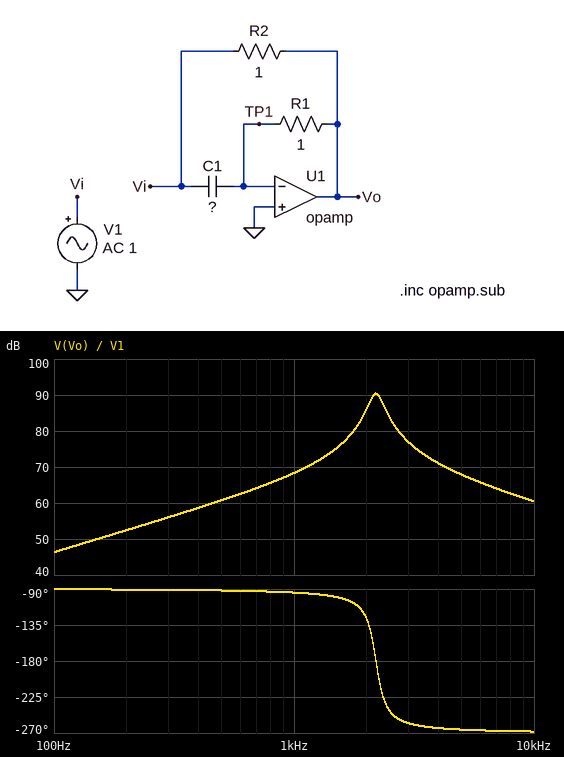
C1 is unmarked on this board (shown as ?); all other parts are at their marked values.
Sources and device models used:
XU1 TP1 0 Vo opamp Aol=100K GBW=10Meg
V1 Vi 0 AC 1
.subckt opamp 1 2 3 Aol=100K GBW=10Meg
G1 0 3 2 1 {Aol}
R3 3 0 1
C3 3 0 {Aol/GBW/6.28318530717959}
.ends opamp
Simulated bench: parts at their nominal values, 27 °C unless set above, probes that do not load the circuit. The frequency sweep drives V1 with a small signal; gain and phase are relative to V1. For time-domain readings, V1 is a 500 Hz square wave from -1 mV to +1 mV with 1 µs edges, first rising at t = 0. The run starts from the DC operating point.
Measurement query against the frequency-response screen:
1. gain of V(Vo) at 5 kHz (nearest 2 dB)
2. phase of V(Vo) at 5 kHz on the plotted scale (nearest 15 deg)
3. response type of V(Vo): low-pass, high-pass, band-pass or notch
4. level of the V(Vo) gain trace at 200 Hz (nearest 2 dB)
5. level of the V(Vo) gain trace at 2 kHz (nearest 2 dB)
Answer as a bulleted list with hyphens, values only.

- 68 dB
- -270 deg
- band-pass
- 52 dB
- 86 dB
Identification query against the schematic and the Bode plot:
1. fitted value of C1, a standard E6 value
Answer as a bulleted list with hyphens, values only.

- 330 mF
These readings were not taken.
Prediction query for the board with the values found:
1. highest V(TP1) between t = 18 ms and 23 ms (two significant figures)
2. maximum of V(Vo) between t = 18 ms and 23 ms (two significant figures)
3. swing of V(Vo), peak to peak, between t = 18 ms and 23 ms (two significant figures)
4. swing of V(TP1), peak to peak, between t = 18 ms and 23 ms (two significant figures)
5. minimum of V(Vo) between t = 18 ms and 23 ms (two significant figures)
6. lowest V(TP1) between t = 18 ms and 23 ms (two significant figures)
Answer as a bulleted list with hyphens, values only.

- 1.6 mV
- 6.7 V
- 13 V
- 3.3 mV
- -6.7 V
- -1.6 mV
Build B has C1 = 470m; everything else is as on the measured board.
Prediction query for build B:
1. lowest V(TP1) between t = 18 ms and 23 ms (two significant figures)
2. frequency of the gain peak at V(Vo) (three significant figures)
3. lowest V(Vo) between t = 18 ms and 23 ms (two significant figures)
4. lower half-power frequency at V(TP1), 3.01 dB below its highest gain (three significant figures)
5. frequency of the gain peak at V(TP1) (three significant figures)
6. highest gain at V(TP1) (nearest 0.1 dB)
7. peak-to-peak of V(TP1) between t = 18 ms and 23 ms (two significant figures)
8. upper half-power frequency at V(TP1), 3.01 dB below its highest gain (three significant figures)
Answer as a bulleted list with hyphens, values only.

- -1.6 mV
- 1.84 kHz
- -7.9 V
- 1.72 kHz
- 1.85 kHz
- 15.9 dB
- 3.2 mV
- 2.03 kHz
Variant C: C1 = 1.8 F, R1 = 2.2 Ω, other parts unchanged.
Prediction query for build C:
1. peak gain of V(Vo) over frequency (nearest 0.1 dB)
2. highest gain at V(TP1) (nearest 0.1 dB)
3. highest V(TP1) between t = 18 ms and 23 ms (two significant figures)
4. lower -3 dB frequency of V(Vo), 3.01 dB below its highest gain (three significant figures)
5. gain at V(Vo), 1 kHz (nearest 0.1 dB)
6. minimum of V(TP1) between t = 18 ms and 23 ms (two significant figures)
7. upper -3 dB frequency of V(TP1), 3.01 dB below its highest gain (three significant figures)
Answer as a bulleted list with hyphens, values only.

- 92.2 dB
- 9.0 dB
- 2.7 mV
- 523 Hz
- 83.8 dB
- -2.7 mV
- 844 Hz
